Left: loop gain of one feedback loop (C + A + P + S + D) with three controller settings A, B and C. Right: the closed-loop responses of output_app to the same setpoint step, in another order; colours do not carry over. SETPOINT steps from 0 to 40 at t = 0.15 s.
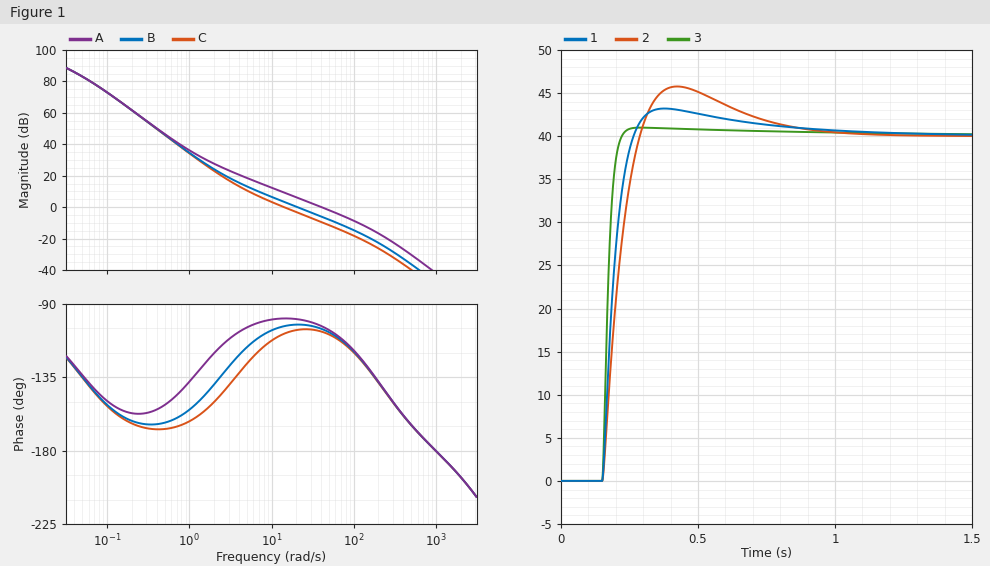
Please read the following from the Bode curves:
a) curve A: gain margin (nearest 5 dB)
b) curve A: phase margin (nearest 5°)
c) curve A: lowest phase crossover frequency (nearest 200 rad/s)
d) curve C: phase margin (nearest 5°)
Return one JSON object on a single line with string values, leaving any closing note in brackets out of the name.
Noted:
{"curve A: gain margin": "40 dB", "curve A: phase margin": "75°", "curve A: lowest phase crossover frequency": "1000 rad/s", "curve C: phase margin": "70°"}
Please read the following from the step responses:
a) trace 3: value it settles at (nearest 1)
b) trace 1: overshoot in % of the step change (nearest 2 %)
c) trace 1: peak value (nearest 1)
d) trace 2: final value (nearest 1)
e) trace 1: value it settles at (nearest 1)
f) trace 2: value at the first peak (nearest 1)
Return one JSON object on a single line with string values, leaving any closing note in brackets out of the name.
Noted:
{"trace 3: value it settles at": "40", "trace 1: overshoot in % of the step change": "8 %", "trace 1: peak value": "43", "trace 2: final value": "40", "trace 1: value it settles at": "40", "trace 2: value at the first peak": "46"}
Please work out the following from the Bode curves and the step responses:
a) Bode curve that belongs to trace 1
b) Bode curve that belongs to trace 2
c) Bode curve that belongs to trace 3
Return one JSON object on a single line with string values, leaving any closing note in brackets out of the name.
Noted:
{"Bode curve that belongs to trace 1": "B", "Bode curve that belongs to trace 2": "C", "Bode curve that belongs to trace 3": "A"}
